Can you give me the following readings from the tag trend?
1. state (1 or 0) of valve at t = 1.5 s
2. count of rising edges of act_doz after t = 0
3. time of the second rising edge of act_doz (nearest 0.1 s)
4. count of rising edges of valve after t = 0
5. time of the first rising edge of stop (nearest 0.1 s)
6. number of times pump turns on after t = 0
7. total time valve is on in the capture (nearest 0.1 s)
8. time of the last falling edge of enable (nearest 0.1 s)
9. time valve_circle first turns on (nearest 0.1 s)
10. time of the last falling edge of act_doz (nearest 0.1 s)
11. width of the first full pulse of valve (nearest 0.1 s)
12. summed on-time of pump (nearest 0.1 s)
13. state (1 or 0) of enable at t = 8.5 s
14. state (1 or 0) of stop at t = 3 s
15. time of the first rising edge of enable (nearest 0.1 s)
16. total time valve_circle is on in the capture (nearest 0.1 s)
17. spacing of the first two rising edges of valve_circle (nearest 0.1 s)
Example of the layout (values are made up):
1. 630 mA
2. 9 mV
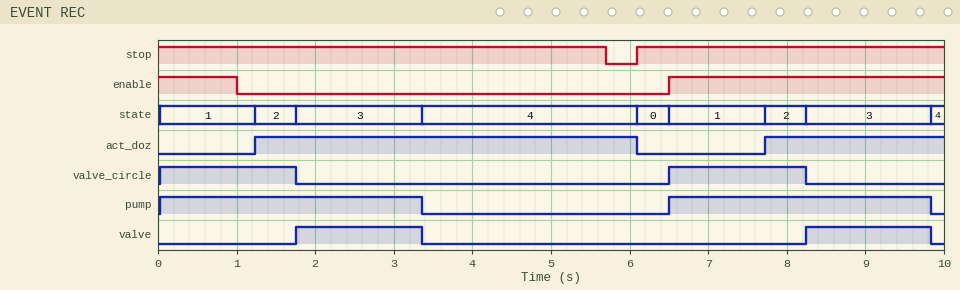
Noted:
1. 0
2. 2
3. 7.7 s
4. 2
5. 6.1 s
6. 2
7. 3.2 s
8. 1.0 s
9. 0.0 s
10. 6.1 s
11. 1.6 s
12. 6.7 s
13. 1
14. 1
15. 6.5 s
16. 3.5 s
17. 6.5 s
